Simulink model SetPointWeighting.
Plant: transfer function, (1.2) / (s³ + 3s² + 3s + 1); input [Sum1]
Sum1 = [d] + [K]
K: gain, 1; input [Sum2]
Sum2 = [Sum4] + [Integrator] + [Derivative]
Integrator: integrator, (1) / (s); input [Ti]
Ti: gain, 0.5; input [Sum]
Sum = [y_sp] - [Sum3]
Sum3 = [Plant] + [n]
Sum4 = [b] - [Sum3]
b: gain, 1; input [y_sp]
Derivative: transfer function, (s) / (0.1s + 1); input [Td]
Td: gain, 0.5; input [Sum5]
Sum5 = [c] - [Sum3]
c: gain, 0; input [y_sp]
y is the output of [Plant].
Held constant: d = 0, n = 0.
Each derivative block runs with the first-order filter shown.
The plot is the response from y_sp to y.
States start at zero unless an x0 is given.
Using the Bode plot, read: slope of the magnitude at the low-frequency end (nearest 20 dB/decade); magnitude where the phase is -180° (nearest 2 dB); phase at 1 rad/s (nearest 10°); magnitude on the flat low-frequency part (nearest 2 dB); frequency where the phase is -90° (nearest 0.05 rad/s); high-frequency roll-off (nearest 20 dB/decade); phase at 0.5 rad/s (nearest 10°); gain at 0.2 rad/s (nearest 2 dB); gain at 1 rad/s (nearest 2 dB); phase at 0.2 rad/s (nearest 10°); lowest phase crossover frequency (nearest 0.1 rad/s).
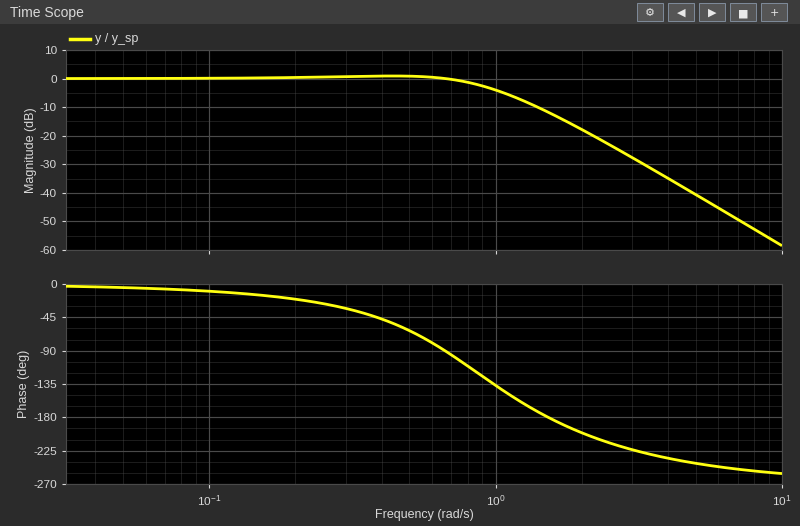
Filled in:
0 dB/decade
-12 dB
-140°
0 dB
0.65 rad/s
-60 dB/decade
-60°
0 dB
-4 dB
-20°
1.5 rad/s
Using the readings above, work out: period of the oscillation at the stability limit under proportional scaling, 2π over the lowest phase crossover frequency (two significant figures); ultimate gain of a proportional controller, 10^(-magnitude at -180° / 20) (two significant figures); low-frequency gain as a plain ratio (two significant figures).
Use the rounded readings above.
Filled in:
4.2 s
4.0
1.0
